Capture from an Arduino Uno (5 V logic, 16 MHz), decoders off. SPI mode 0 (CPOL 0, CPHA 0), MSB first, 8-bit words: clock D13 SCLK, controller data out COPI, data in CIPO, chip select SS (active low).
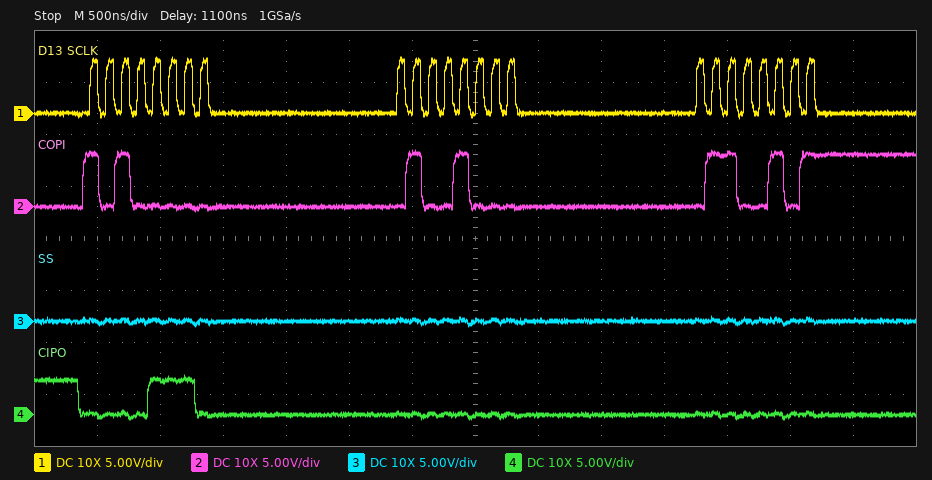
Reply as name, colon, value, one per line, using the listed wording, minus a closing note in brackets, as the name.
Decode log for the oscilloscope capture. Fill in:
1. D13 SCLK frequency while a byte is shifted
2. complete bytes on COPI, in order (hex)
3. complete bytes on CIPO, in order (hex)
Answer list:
D13 SCLK frequency while a byte is shifted: 8 MHz
complete bytes on COPI, in order: A0 48 65
complete bytes on CIPO, in order: 0E 00 00
